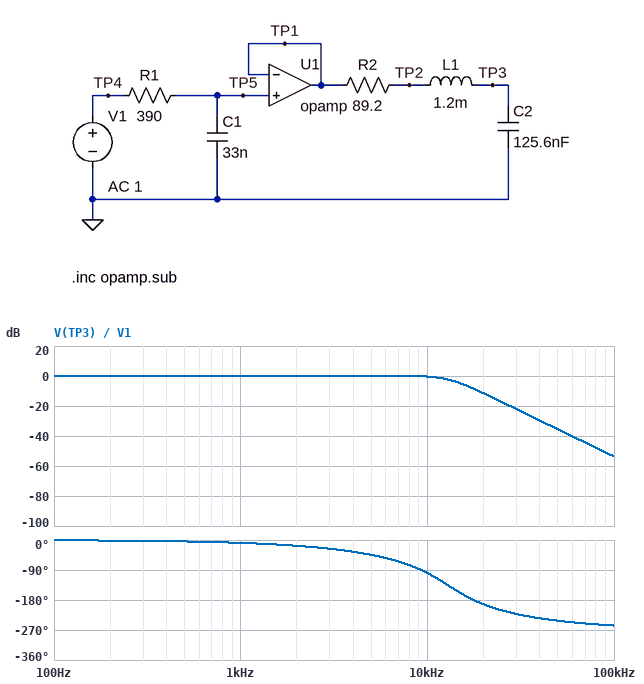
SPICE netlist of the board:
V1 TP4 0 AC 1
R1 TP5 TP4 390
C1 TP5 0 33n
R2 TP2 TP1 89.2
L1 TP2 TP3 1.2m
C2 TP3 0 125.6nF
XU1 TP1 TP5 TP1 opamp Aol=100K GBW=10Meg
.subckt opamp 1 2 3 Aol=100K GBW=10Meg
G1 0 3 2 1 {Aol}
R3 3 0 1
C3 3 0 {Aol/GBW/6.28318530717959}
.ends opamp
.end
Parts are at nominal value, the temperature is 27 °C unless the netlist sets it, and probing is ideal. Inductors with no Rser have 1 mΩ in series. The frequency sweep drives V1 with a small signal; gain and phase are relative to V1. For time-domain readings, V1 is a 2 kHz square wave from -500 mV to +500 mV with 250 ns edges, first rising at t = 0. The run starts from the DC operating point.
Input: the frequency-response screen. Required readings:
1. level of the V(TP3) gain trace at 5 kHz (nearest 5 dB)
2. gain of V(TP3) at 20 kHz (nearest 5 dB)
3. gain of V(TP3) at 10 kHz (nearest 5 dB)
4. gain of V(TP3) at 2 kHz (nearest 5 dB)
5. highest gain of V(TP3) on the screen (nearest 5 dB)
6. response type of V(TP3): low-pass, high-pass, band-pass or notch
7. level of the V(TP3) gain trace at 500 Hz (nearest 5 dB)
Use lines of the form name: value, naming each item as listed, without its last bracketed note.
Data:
level of the V(TP3) gain trace at 5 kHz: 0 dB
gain of V(TP3) at 20 kHz: -10 dB
gain of V(TP3) at 10 kHz: 0 dB
gain of V(TP3) at 2 kHz: 0 dB
highest gain of V(TP3) on the screen: 0 dB
response type of V(TP3): low-pass, high-pass, band-pass or notch: low-pass
level of the V(TP3) gain trace at 500 Hz: 0 dB
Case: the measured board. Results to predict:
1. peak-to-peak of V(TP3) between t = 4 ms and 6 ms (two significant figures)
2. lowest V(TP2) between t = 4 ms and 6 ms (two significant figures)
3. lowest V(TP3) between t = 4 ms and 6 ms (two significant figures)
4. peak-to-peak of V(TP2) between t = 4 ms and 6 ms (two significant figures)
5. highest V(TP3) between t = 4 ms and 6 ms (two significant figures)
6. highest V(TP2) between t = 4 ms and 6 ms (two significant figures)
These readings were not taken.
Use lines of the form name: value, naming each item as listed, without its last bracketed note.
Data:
peak-to-peak of V(TP3) between t = 4 ms and 6 ms: 1.2 V
lowest V(TP2) between t = 4 ms and 6 ms: -550 mV
lowest V(TP3) between t = 4 ms and 6 ms: -600 mV
peak-to-peak of V(TP2) between t = 4 ms and 6 ms: 1.1 V
highest V(TP3) between t = 4 ms and 6 ms: 600 mV
highest V(TP2) between t = 4 ms and 6 ms: 550 mV
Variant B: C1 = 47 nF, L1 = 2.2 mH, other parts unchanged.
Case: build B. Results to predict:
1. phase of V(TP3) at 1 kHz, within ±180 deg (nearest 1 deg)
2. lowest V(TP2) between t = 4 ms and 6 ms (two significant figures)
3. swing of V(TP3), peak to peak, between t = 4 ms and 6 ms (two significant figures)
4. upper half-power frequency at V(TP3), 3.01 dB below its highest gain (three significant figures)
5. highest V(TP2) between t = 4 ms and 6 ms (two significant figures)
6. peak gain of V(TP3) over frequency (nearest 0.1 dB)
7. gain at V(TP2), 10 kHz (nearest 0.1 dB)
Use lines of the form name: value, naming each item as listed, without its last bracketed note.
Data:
phase of V(TP3) at 1 kHz, within ±180 deg: -11 deg
lowest V(TP2) between t = 4 ms and 6 ms: -570 mV
swing of V(TP3), peak to peak, between t = 4 ms and 6 ms: 1.3 V
upper half-power frequency at V(TP3), 3.01 dB below its highest gain: 10.6 kHz
highest V(TP2) between t = 4 ms and 6 ms: 570 mV
peak gain of V(TP3) over frequency: 1.3 dB
gain at V(TP2), 10 kHz: -21.5 dB
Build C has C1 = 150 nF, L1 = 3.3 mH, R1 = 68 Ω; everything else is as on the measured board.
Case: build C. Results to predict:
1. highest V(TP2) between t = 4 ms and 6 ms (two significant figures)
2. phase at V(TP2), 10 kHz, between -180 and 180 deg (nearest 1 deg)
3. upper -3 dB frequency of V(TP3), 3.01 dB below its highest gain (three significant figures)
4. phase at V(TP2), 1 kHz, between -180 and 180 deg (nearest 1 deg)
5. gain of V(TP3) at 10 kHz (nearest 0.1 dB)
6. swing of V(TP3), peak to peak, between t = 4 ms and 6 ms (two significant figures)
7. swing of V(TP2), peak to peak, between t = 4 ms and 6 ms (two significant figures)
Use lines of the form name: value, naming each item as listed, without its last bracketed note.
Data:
highest V(TP2) between t = 4 ms and 6 ms: 630 mV
phase at V(TP2), 10 kHz, between -180 and 180 deg: 15 deg
upper -3 dB frequency of V(TP3), 3.01 dB below its highest gain: 9.00 kHz
phase at V(TP2), 1 kHz, between -180 and 180 deg: -8 deg
gain of V(TP3) at 10 kHz: -1.0 dB
swing of V(TP3), peak to peak, between t = 4 ms and 6 ms: 1.7 V
swing of V(TP2), peak to peak, between t = 4 ms and 6 ms: 1.3 V
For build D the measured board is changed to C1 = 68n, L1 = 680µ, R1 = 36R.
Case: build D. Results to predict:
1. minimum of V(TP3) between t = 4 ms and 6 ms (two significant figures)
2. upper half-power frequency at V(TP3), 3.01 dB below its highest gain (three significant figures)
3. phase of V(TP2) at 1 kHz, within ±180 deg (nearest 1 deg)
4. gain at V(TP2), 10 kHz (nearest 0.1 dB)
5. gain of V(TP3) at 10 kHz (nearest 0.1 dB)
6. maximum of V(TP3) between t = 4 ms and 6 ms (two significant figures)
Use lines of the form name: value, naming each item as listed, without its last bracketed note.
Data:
minimum of V(TP3) between t = 4 ms and 6 ms: -590 mV
upper half-power frequency at V(TP3), 3.01 dB below its highest gain: 18.6 kHz
phase of V(TP2) at 1 kHz, within ±180 deg: -5 deg
gain at V(TP2), 10 kHz: -3.4 dB
gain of V(TP3) at 10 kHz: 0.2 dB
maximum of V(TP3) between t = 4 ms and 6 ms: 590 mV
